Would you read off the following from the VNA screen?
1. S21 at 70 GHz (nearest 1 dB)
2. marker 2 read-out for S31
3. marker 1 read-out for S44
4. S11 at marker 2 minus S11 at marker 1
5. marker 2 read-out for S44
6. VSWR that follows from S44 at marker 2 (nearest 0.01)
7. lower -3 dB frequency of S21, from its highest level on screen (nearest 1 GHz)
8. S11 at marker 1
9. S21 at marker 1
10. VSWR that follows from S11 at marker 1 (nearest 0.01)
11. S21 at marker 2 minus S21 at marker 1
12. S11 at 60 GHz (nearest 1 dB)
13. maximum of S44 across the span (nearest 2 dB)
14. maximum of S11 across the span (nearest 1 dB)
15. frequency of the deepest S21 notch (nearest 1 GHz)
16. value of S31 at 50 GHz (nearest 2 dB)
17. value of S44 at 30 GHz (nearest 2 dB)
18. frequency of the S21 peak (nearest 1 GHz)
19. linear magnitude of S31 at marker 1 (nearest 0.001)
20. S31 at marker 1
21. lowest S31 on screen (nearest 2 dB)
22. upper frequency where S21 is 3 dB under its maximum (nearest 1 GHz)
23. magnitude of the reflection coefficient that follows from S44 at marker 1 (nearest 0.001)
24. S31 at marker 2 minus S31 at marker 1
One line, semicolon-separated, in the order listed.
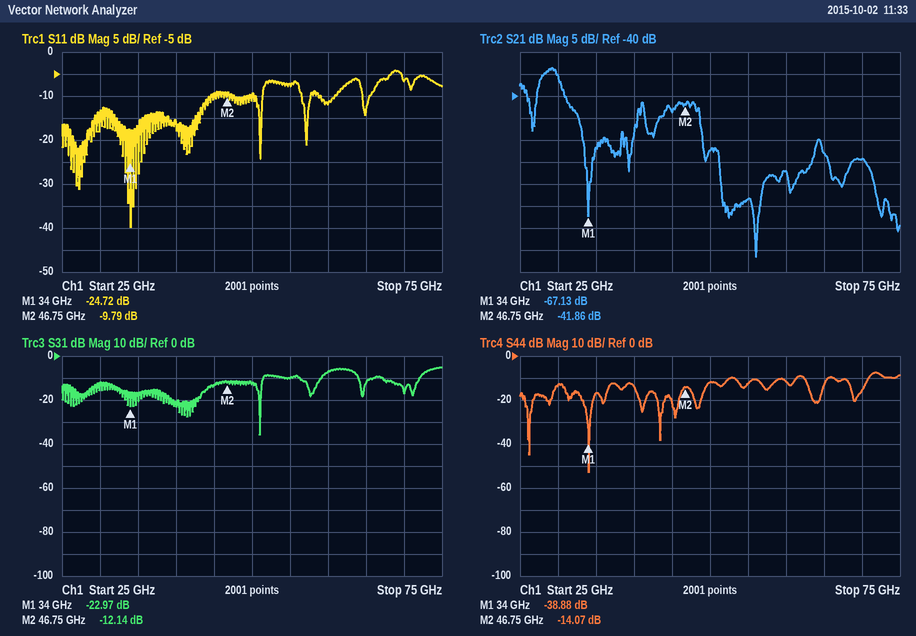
-54 dB; -12.14 dB; -38.88 dB; 14.93 dB; -14.07 dB; 1.49; 28 GHz; -24.72 dB; -67.13 dB; 1.12; 25.27 dB; -12 dB; -8 dB; -4 dB; 56 GHz; -12 dB; -14 dB; 29 GHz; 0.071; -22.97 dB; -36 dB; 30 GHz; 0.011; 10.83 dB
